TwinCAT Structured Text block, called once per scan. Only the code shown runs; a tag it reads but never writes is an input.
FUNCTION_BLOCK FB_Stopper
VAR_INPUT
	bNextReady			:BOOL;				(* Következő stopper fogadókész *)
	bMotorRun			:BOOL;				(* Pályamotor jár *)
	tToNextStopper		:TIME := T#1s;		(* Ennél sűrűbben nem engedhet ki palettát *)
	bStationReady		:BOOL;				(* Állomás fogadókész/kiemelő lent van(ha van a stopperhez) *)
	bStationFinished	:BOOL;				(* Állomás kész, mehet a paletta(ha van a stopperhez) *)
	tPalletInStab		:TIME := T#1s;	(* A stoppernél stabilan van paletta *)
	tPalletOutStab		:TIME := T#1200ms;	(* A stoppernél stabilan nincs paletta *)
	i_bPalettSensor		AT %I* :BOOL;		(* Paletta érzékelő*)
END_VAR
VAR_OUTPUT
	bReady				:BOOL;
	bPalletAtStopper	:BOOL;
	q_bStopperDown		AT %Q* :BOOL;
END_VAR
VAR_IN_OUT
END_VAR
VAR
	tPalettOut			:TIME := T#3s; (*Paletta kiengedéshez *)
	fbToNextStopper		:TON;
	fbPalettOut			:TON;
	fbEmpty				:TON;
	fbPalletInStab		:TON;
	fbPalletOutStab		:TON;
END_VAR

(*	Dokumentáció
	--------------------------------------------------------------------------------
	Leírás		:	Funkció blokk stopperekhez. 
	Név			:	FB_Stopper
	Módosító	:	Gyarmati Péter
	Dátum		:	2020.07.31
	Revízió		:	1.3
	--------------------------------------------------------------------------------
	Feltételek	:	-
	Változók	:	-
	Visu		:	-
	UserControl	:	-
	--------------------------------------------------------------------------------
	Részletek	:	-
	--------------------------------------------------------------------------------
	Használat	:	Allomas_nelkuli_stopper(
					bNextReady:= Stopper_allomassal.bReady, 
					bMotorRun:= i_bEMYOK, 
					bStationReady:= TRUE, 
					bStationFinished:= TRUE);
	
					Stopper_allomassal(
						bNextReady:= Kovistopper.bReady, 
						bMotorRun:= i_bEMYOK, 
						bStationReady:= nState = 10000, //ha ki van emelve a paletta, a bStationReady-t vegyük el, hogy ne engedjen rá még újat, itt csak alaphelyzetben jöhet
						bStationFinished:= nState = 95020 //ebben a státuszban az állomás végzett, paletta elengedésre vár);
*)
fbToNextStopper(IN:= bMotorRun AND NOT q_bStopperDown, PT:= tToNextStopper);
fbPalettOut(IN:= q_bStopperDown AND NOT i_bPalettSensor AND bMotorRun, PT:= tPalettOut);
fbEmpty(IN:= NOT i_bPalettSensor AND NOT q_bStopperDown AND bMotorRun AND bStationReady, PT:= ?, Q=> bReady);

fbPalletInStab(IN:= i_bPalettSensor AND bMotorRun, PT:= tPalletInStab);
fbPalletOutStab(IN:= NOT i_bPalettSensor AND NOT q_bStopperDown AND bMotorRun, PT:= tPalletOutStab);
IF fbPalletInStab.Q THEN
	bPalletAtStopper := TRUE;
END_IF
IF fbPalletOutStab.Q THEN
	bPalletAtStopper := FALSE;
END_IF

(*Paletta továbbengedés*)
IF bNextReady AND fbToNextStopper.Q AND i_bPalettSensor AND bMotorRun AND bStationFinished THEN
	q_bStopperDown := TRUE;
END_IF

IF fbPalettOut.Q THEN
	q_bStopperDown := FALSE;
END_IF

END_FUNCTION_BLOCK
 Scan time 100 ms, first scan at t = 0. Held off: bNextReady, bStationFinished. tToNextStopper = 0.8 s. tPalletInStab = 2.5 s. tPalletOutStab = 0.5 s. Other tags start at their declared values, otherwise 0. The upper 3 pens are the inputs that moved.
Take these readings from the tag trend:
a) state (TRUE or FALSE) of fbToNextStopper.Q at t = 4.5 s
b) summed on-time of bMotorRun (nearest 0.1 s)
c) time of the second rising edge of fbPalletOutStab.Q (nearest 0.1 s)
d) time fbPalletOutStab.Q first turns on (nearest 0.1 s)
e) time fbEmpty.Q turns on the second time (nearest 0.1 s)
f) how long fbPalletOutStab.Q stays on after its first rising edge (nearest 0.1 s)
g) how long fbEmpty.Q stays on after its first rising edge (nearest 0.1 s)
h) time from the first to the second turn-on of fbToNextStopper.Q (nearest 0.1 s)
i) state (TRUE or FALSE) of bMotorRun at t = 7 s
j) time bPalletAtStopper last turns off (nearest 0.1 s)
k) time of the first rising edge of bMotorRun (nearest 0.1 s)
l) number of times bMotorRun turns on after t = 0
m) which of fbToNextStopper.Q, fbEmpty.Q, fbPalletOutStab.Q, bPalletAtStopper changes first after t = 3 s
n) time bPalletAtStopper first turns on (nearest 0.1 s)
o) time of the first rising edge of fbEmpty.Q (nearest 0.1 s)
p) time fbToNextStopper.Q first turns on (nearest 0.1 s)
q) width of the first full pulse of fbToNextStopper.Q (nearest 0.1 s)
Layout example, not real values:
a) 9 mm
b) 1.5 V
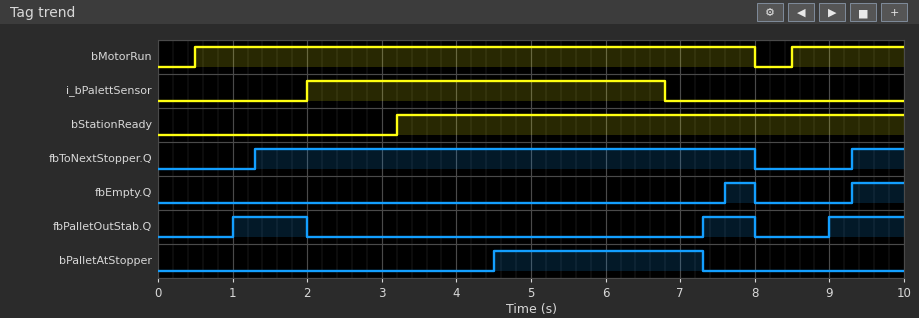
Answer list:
a) TRUE
b) 9.0 s
c) 7.3 s
d) 1.0 s
e) 9.3 s
f) 1.0 s
g) 0.4 s
h) 8.0 s
i) TRUE
j) 7.3 s
k) 0.5 s
l) 2
m) bPalletAtStopper
n) 4.5 s
o) 7.6 s
p) 1.3 s
q) 6.7 s
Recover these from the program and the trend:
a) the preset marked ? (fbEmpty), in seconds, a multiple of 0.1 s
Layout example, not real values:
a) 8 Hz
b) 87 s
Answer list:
a) 0.8 s
